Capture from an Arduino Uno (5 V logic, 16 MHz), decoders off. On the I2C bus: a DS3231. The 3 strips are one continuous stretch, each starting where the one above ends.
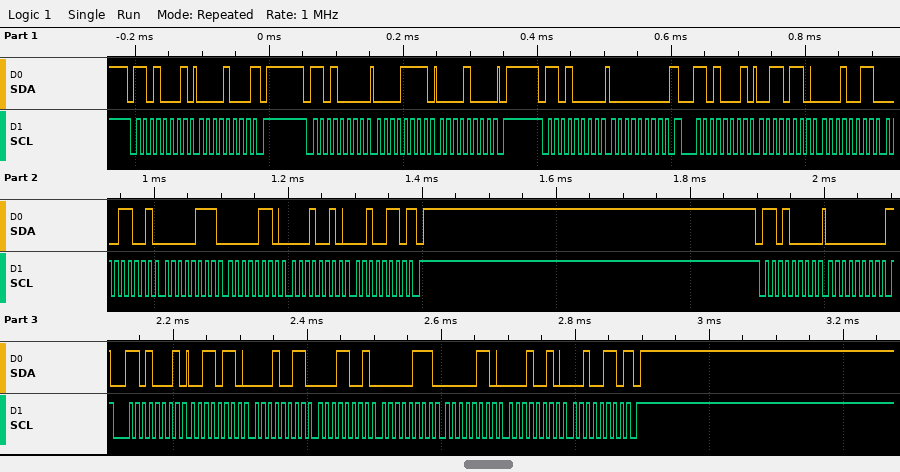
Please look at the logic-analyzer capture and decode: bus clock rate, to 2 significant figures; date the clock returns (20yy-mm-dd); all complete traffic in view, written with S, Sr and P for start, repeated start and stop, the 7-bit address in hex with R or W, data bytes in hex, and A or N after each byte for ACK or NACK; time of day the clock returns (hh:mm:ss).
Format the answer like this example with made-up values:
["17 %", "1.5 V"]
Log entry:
["100 kHz", "2026-12-06", "S 68R A 08 N P S 68W A 0F A 08 A P S 68W A 00 A Sr 68R A 36 A 13 A 19 A 07 A 06 A 12 A 26 N P S 68W A 00 A Sr 68R A 36 A 13 A 19 A 07 A 06 A 12 A 26 N P", "19:13:36"]
